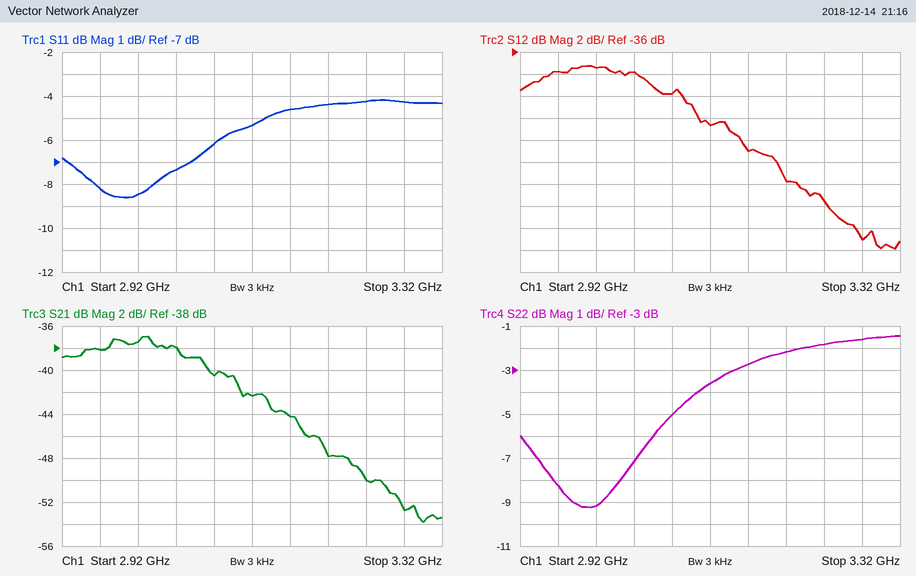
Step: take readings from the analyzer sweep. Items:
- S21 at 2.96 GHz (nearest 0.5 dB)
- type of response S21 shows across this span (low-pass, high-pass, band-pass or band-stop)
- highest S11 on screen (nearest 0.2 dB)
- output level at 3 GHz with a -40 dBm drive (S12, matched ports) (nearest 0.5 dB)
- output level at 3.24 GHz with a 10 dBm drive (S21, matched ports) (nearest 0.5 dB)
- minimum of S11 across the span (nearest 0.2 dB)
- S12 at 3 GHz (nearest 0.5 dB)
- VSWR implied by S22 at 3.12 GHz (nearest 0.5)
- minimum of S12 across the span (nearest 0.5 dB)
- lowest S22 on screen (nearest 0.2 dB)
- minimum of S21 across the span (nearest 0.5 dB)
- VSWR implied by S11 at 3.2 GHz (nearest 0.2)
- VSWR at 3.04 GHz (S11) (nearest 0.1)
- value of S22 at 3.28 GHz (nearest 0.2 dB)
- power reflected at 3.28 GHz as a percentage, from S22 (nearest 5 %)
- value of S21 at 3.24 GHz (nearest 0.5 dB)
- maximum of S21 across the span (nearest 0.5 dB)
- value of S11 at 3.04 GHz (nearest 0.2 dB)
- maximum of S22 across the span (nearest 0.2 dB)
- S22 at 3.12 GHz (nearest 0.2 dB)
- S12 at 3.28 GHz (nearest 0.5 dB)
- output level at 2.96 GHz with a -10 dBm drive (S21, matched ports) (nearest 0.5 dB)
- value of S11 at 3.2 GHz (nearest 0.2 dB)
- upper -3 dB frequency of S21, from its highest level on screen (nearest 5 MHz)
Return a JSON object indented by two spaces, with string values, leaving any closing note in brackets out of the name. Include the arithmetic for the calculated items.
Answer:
{
  "S21 at 2.96 GHz": "-38.0 dB",
  "type of response S21 shows across this span": "low-pass",
  "highest S11 on screen": "-4.2 dB",
  "output level at 3 GHz with a -40 dBm drive (S12, matched ports)": "-40 dBm + (-37.5 dB) = -77.5 dBm",
  "output level at 3.24 GHz with a 10 dBm drive (S21, matched ports)": "10 dBm + (-50.0 dB) = -40.0 dBm",
  "minimum of S11 across the span": "-8.6 dB",
  "S12 at 3 GHz": "-37.5 dB",
  "VSWR implied by S22 at 3.12 GHz": "|Γ| = 10^(-3.6/20) = 0.6607; VSWR = (1 + 0.6607)/(1 − 0.6607) ≈ 4.89, so 5.0 to the nearest 0.5",
  "minimum of S12 across the span": "-54.0 dB",
  "lowest S22 on screen": "-9.2 dB",
  "minimum of S21 across the span": "-54.0 dB",
  "VSWR implied by S11 at 3.2 GHz": "|Γ| = 10^(-4.4/20) = 0.6026; VSWR = (1 + 0.6026)/(1 − 0.6026) ≈ 4.0",
  "VSWR at 3.04 GHz (S11)": "|Γ| = 10^(-7.4/20) = 0.4266; VSWR = (1 + 0.4266)/(1 − 0.4266) ≈ 2.5",
  "value of S22 at 3.28 GHz": "-1.6 dB",
  "power reflected at 3.28 GHz as a percentage, from S22": "10^(-1.6/10) ≈ 69.2 %, so 70 % to the nearest 5 %",
  "value of S21 at 3.24 GHz": "-50.0 dB",
  "maximum of S21 across the span": "-37.0 dB",
  "value of S11 at 3.04 GHz": "-7.4 dB",
  "maximum of S22 across the span": "-1.4 dB",
  "S22 at 3.12 GHz": "-3.6 dB",
  "S12 at 3.28 GHz": "-53.0 dB",
  "output level at 2.96 GHz with a -10 dBm drive (S21, matched ports)": "-10 dBm + (-38.0 dB) = -48.0 dBm",
  "value of S11 at 3.2 GHz": "-4.4 dB",
  "upper -3 dB frequency of S21, from its highest level on screen": "3.075 GHz"
}
